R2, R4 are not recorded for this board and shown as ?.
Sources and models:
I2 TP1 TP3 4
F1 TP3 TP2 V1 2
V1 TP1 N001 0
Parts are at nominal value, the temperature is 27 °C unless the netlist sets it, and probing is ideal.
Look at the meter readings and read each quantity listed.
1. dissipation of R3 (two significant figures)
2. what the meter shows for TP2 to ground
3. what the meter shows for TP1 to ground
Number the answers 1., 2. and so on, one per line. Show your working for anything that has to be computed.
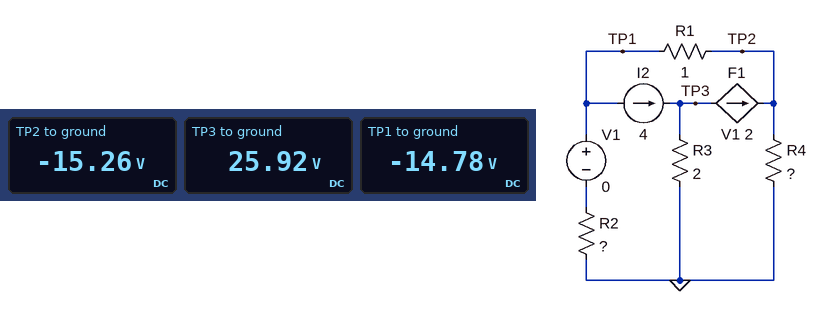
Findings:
1. (25.92 V)^2 / 2 Ω = 340 W
2. -15.26 V
3. -14.78 V
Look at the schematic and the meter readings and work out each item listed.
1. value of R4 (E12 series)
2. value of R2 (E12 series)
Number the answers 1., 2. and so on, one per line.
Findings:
1. 1.8 Ω
2. 3.3 Ω
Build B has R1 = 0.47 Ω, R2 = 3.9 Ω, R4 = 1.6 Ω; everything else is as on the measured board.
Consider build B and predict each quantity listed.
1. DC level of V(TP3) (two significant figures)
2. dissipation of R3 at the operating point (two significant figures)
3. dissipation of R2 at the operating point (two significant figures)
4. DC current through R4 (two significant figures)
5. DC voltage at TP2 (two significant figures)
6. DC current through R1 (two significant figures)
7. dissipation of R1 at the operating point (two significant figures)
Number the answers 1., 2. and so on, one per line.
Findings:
1. 20 V
2. 200 W
3. 35 W
4. 7.0 A
5. -11 V
6. 1.0 A
7. 480 mW
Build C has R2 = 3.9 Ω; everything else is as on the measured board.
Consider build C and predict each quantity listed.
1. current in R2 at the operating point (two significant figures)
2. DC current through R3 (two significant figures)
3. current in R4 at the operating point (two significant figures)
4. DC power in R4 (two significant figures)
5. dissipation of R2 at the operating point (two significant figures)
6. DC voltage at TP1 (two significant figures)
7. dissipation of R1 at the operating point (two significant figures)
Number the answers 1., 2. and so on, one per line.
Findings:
1. 3.6 A
2. 11 A
3. 7.6 A
4. 100 W
5. 51 W
6. -14 V
7. 150 mW
